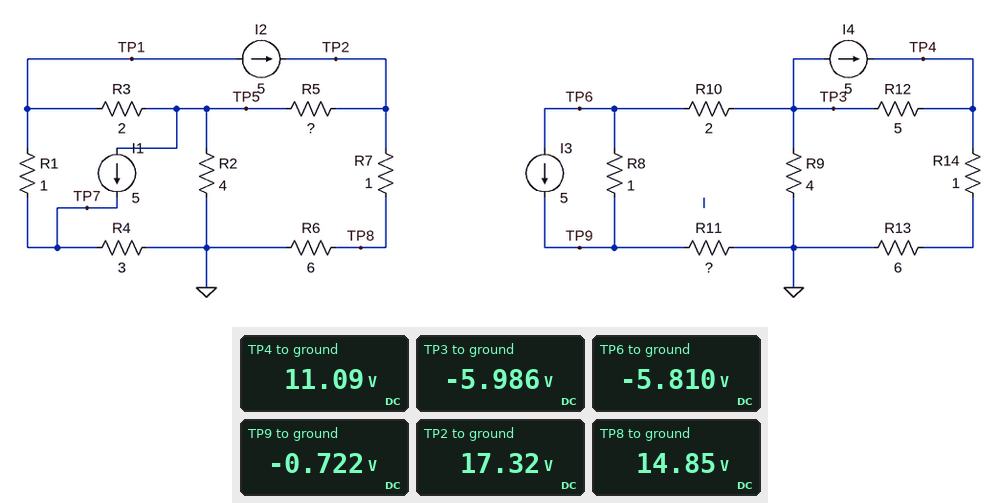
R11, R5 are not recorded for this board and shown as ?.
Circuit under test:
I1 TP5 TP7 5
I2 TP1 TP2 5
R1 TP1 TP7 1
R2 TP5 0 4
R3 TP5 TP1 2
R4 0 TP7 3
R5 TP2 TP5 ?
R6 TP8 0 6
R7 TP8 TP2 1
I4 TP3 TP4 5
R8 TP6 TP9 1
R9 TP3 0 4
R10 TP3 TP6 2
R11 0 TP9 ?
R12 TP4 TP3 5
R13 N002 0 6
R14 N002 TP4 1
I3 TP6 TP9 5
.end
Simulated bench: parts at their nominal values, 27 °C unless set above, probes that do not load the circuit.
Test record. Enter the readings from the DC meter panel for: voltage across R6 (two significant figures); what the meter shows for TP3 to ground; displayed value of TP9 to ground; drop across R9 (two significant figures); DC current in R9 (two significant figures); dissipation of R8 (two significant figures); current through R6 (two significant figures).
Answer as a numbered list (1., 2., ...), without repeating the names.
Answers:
1. 15 V
2. -5.986 V
3. -0.722 V
4. 6.0 V
5. 1.5 A
6. 26 W
7. 2.5 A
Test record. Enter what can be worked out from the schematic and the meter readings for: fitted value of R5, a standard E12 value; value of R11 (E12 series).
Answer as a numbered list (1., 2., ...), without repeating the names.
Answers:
1. 10 Ω
2. 8.2 Ω
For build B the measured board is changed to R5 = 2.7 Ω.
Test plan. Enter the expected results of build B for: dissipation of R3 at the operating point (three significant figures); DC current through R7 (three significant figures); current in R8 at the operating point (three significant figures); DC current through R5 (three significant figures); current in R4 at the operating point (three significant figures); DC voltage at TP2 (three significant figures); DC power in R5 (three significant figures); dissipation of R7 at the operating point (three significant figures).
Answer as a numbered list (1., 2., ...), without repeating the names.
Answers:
1. 28.7 mW
2. 950 mA
3. 5.09 A
4. 4.05 A
5. 120 mA
6. 6.65 V
7. 44.3 W
8. 903 mW
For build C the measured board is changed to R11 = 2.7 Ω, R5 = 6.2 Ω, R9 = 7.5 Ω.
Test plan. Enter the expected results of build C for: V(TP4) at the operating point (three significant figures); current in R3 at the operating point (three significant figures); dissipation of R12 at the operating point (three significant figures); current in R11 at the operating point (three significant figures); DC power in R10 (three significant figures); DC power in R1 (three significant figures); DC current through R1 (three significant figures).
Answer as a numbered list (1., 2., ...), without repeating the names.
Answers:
1. 10.2 V
2. 244 mA
3. 62.9 W
4. 447 mA
5. 400 mW
6. 27.5 W
7. 5.24 A
